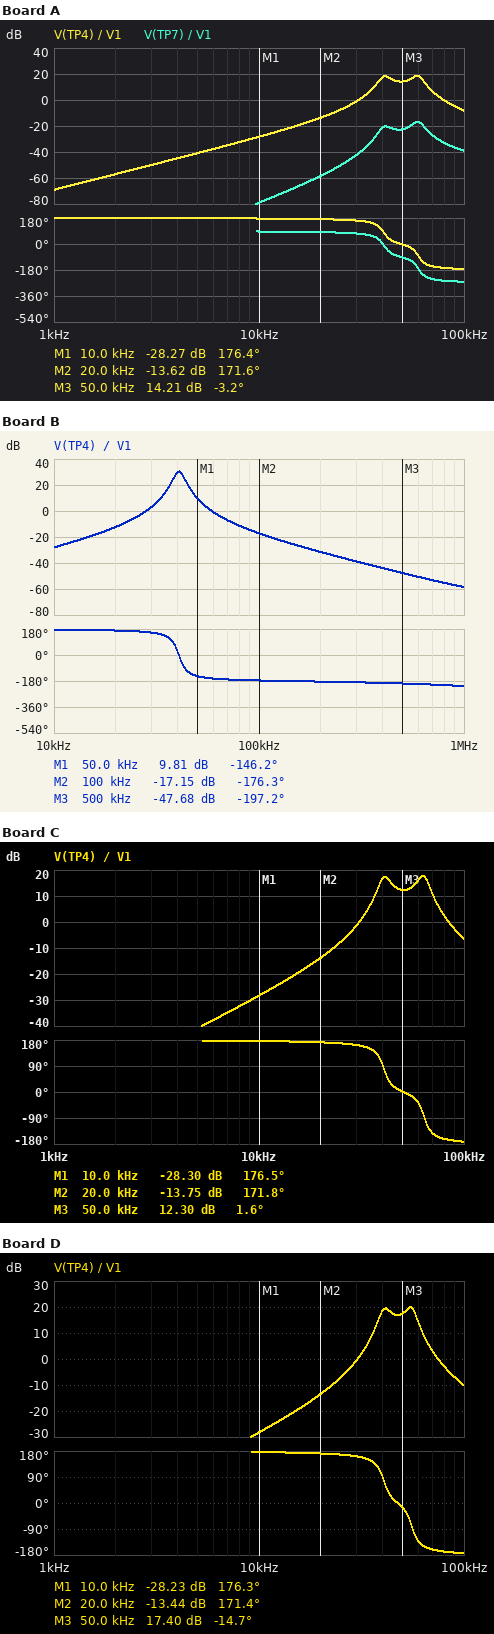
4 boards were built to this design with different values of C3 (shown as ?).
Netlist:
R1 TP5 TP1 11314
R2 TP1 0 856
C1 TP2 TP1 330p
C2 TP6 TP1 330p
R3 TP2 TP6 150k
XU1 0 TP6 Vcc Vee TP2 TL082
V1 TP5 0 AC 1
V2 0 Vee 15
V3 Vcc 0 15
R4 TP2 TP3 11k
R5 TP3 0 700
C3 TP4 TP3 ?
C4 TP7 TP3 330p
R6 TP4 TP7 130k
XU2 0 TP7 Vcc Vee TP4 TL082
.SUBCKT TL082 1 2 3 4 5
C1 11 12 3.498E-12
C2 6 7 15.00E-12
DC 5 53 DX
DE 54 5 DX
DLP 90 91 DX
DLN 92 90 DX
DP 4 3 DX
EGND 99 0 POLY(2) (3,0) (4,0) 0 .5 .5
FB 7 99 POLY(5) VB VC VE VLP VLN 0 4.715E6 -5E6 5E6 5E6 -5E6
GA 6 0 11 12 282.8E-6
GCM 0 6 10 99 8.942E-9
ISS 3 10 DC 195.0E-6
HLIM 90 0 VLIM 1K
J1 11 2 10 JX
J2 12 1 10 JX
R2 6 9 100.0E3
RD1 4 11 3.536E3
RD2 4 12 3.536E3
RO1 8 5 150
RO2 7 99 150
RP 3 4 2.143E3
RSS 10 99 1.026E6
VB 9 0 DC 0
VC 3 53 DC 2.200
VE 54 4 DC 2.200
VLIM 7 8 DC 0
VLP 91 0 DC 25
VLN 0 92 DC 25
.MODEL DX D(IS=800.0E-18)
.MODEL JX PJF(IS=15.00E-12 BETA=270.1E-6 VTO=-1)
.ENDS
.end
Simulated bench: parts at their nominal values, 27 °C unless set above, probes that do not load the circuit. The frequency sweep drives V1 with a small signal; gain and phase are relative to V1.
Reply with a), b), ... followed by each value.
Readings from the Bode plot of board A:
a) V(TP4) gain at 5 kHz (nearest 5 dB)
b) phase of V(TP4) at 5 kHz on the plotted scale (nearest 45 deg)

a) -40 dB
b) 180 deg
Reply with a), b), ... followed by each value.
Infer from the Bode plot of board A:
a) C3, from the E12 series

a) 180 pF
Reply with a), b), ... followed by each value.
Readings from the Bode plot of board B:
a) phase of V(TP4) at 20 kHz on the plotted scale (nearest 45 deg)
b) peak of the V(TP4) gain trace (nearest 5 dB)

a) 180 deg
b) 30 dB
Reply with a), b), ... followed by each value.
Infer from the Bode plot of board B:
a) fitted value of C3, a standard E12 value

a) 470 pF
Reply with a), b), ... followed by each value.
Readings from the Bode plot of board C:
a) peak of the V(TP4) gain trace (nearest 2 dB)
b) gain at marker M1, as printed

a) 18 dB
b) -28.30 dB
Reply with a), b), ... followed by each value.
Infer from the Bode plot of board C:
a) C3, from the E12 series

a) 150 pF
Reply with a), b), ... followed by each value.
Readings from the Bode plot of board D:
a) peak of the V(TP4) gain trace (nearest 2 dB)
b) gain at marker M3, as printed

a) 20 dB
b) 17.40 dB
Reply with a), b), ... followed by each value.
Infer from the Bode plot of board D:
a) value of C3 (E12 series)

a) 220 pF
